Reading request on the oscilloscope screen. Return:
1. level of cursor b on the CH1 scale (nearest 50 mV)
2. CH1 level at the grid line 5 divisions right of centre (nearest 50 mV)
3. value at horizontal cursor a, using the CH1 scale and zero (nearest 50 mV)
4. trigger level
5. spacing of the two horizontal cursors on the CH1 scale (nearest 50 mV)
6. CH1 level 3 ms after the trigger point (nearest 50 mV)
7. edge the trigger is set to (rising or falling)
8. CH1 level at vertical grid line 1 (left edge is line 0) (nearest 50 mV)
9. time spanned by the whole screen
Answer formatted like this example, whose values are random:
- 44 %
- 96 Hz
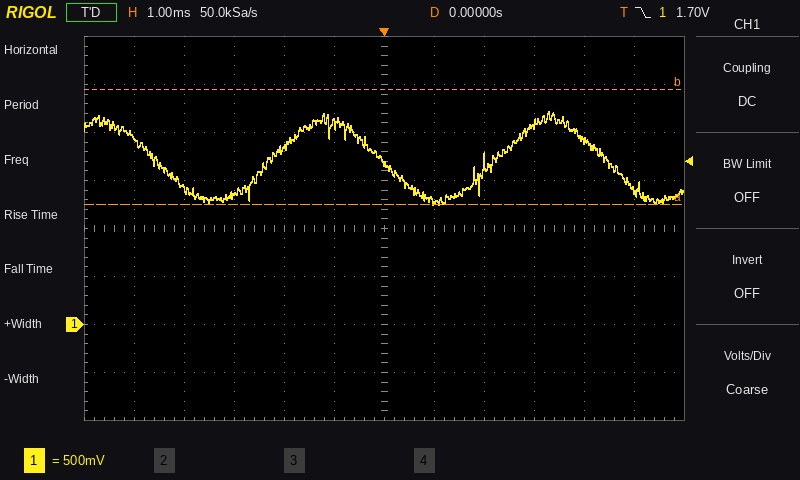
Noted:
- 2.45 V
- 1.40 V
- 1.25 V
- 1.70 V
- 1.20 V
- 2.10 V
- falling
- 1.95 V
- 12 ms
